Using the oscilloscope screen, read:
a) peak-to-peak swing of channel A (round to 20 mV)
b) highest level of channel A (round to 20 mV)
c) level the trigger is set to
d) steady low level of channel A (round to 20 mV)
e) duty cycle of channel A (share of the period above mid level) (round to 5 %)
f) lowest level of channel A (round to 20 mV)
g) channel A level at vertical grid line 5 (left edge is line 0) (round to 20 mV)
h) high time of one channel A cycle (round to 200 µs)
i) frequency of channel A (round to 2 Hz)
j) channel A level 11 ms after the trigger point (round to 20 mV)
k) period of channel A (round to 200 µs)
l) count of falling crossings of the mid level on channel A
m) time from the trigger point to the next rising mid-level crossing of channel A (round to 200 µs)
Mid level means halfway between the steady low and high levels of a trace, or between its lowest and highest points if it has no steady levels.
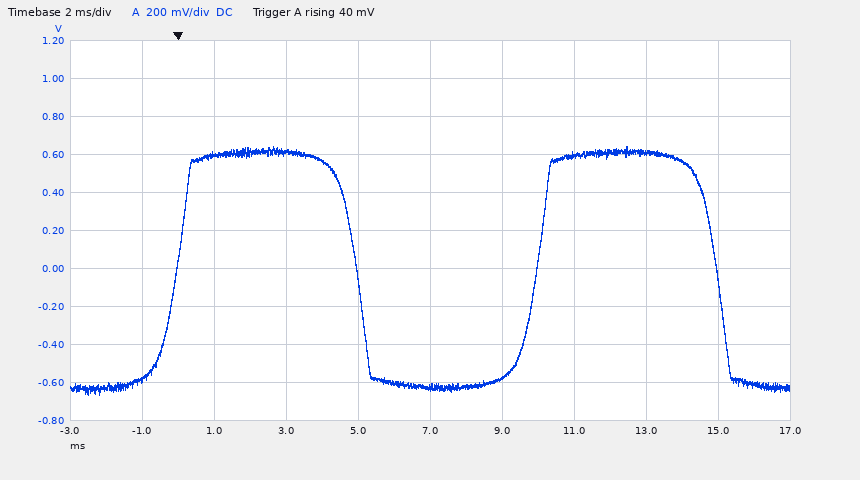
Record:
1.30 V
640 mV
40 mV
-620 mV
50 %
-660 mV
-620 mV
5.0 ms
100 Hz
600 mV
10.0 ms
2
10.0 ms
